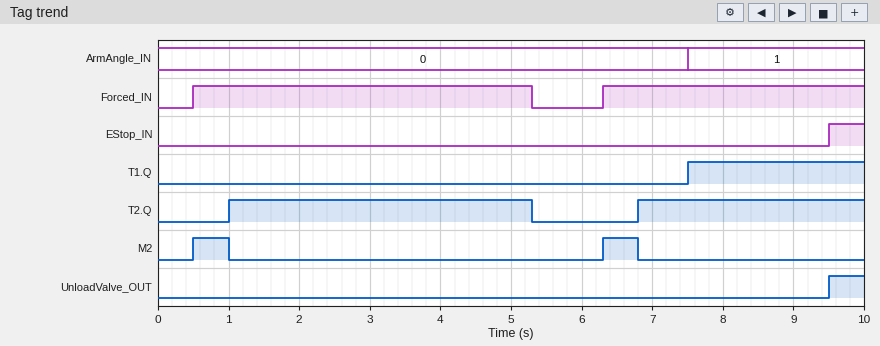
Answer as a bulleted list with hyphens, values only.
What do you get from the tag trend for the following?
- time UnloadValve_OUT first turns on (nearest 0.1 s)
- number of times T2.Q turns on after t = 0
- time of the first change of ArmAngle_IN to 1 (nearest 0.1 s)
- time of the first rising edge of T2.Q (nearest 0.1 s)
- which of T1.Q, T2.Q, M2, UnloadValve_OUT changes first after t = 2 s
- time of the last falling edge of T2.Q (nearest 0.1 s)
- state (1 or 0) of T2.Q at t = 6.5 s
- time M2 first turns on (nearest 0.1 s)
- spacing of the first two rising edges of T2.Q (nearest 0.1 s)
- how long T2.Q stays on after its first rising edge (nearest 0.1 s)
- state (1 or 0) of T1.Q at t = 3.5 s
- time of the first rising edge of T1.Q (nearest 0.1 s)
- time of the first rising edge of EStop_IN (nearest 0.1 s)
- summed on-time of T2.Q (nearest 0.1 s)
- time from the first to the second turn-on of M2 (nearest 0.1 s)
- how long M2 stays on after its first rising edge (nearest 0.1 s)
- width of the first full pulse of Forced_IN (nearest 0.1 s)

- 9.5 s
- 2
- 7.5 s
- 1.0 s
- T2.Q
- 5.3 s
- 0
- 0.5 s
- 5.8 s
- 4.3 s
- 0
- 7.5 s
- 9.5 s
- 7.5 s
- 5.8 s
- 0.5 s
- 4.8 s
